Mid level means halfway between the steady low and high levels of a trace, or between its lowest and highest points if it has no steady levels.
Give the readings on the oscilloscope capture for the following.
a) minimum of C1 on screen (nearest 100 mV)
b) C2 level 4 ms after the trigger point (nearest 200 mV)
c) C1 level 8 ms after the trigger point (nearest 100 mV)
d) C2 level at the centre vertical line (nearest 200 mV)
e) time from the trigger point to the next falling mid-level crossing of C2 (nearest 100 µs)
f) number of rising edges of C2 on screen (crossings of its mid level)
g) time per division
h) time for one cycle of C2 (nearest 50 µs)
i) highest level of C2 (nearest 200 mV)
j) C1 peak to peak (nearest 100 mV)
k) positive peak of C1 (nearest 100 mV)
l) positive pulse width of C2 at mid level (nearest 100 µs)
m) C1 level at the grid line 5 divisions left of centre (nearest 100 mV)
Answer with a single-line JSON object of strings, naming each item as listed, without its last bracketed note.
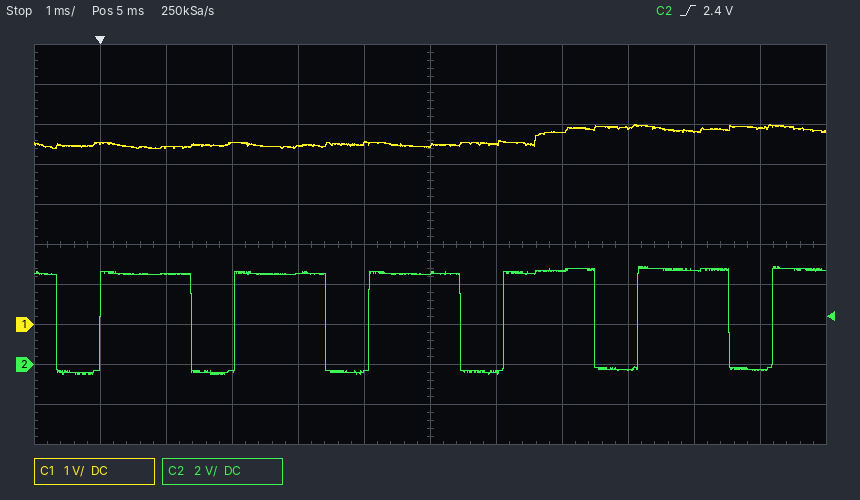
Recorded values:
{"minimum of C1 on screen": "4.4 V", "C2 level 4 ms after the trigger point": "-400 mV", "C1 level 8 ms after the trigger point": "4.9 V", "C2 level at the centre vertical line": "4.6 V", "time from the trigger point to the next falling mid-level crossing of C2": "1.4 ms", "number of rising edges of C2 on screen": "6", "time per division": "1 ms", "time for one cycle of C2": "2.05 ms", "highest level of C2": "4.8 V", "C1 peak to peak": "600 mV", "positive peak of C1": "5.0 V", "positive pulse width of C2 at mid level": "1.4 ms", "C1 level at the grid line 5 divisions left of centre": "4.5 V"}
